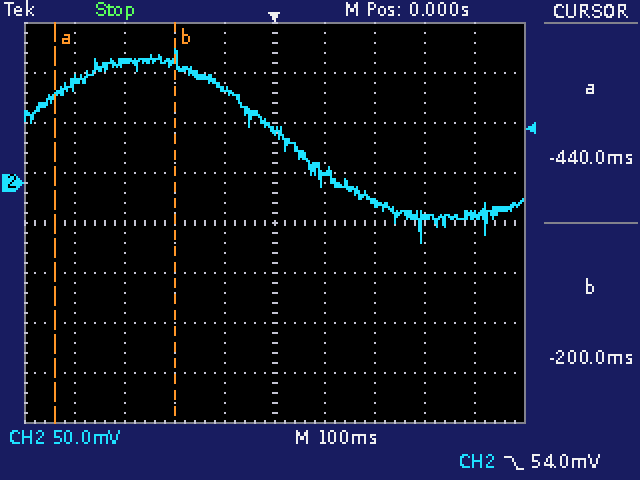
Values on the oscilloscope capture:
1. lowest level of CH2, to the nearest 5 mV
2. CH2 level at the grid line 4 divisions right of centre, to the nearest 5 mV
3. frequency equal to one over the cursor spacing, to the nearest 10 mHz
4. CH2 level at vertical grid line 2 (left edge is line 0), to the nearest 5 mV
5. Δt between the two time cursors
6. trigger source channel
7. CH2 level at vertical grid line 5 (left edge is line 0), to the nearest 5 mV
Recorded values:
-60 mV
-30 mV
4.17 Hz
120 mV
240 ms
CH2
50 mV
